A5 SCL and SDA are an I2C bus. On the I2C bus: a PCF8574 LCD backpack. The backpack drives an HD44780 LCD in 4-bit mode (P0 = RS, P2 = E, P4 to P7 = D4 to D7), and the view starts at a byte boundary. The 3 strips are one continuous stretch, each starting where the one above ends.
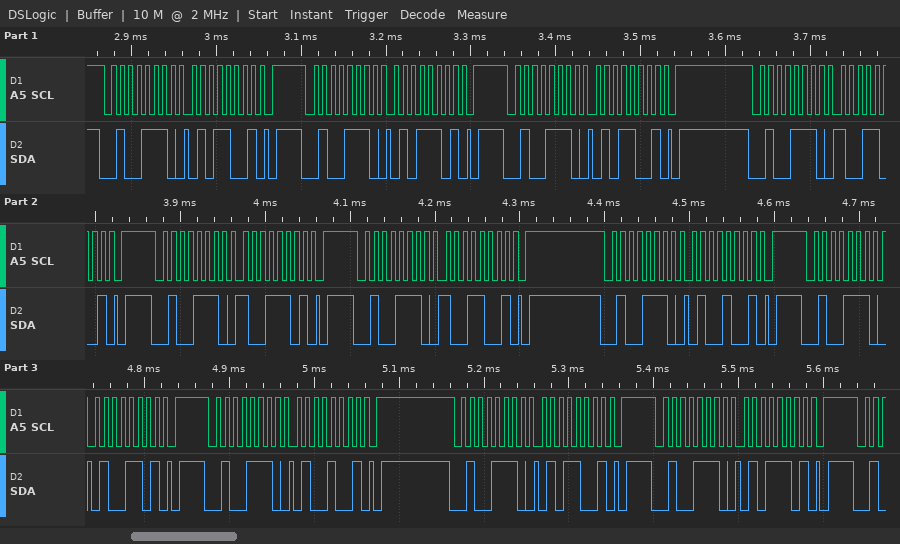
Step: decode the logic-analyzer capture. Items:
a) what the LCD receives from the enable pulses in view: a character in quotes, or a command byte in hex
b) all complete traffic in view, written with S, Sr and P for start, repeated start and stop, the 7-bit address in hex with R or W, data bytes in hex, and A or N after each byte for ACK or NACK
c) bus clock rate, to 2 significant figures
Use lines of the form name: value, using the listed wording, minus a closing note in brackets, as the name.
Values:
what the LCD receives from the enable pulses in view: a character in quotes, or a command byte in hex: 'Y'
all complete traffic in view, written with S, Sr and P for start, repeated start and stop, the 7-bit address in hex with R or W, data bytes in hex, and A or N after each byte for ACK or NACK: S 27W A 59 A P S 27W A 5D A P S 27W A 59 A P S 27W A 99 A P S 27W A 9D A P S 27W A 99 A P S 27W A 49 A P S 27W A 4D A P S 27W A 49 A P S 27W A 59 A P S 27W A 5D A P
bus clock rate, to 2 significant figures: 100 kHz
